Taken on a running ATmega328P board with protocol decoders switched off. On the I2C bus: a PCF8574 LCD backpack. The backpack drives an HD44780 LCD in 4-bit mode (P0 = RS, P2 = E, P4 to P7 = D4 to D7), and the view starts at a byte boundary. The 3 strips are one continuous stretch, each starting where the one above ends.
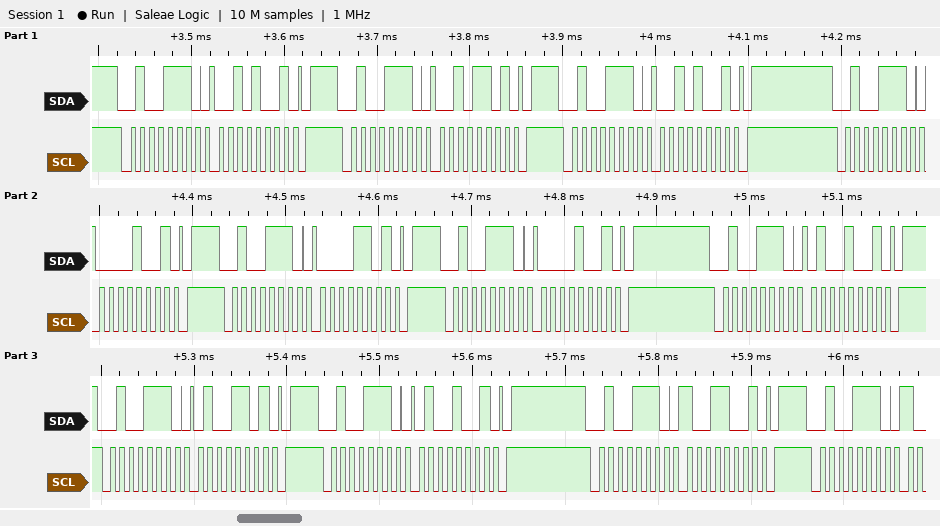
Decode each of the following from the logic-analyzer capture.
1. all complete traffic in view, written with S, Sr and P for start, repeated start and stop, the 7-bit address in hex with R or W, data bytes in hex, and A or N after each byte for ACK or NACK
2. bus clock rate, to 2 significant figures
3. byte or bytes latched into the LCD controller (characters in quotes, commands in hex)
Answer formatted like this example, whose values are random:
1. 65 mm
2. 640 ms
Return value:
1. S 27W A 29 A P S 27W A 2D A P S 27W A 29 A P S 27W A 09 A P S 27W A 0D A P S 27W A 09 A P S 27W A 49 A P S 27W A 4D A P S 27W A 49 A P S 27W A 99 A P S 27W A
2. 100 kHz
3. ' '
